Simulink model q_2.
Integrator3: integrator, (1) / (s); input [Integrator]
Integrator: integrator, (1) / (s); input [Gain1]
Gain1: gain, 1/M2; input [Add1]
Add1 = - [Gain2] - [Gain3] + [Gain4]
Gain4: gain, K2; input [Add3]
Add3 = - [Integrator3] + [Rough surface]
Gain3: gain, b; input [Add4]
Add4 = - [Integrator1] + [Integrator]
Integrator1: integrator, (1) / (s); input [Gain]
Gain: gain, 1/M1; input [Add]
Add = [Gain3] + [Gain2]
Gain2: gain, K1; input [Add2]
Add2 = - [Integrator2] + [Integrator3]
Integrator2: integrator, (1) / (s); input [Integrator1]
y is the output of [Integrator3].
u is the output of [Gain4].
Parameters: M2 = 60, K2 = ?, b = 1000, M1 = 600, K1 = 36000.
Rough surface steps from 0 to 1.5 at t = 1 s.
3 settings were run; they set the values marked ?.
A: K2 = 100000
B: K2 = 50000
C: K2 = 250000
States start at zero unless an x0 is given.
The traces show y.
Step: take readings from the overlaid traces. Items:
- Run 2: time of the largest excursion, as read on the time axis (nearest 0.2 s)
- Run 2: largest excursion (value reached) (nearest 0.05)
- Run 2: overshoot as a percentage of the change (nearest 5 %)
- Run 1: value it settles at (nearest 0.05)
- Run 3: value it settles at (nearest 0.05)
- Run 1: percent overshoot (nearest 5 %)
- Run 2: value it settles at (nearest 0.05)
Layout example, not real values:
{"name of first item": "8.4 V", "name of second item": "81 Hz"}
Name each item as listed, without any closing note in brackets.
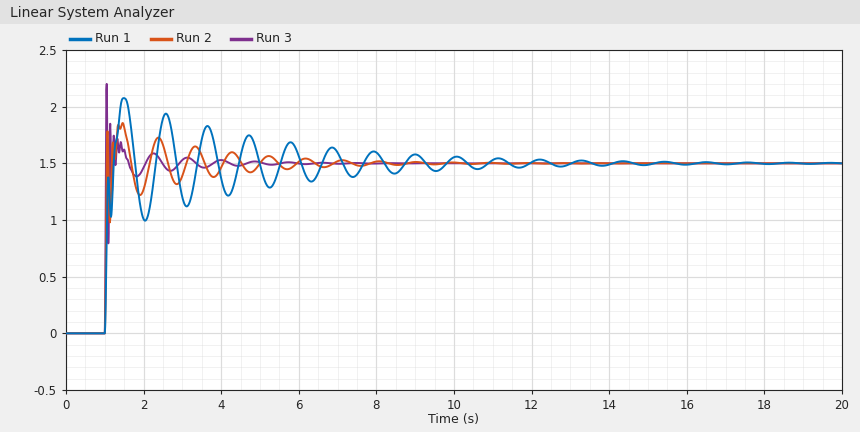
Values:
{"Run 2: time of the largest excursion, as read on the time axis": "1.4 s", "Run 2: largest excursion (value reached)": "1.85", "Run 2: overshoot as a percentage of the change": "25 %", "Run 1: value it settles at": "1.50", "Run 3: value it settles at": "1.50", "Run 1: percent overshoot": "40 %", "Run 2: value it settles at": "1.50"}
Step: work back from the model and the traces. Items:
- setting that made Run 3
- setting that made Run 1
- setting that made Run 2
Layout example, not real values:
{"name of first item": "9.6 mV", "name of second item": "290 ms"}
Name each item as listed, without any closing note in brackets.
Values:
{"setting that made Run 3": "C", "setting that made Run 1": "B", "setting that made Run 2": "A"}
